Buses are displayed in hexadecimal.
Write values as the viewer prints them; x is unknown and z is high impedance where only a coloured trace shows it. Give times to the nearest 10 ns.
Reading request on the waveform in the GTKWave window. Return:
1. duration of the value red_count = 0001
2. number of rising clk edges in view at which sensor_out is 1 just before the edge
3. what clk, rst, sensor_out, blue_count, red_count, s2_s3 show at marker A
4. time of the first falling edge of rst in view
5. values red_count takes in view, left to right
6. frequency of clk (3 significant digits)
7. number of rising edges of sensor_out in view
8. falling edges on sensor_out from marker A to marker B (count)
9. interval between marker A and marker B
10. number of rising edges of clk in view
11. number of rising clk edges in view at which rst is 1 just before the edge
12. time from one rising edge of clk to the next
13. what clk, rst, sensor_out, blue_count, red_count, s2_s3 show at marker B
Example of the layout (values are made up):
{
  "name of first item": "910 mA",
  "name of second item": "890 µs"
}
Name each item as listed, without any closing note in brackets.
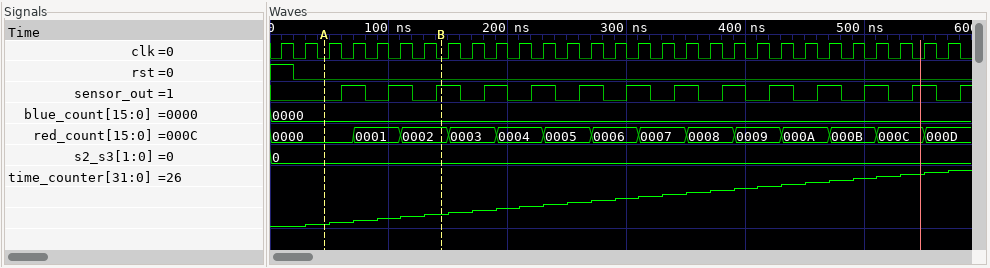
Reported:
{
  "duration of the value red_count = 0001": "40 ns",
  "number of rising clk edges in view at which sensor_out is 1 just before the edge": "13",
  "what clk, rst, sensor_out, blue_count, red_count, s2_s3 show at marker A": "clk=0, rst=0, sensor_out=0, blue_count=0000, red_count=0000, s2_s3=0",
  "time of the first falling edge of rst in view": "20 ns",
  "values red_count takes in view, left to right": "0000, 0001, 0002, 0003, 0004, 0005, 0006, 0007, 0008, 0009, 000A, 000B, 000C, 000D",
  "frequency of clk": "50.0 MHz",
  "number of rising edges of sensor_out in view": "14",
  "falling edges on sensor_out from marker A to marker B": "2",
  "interval between marker A and marker B": "100 ns",
  "number of rising edges of clk in view": "29",
  "number of rising clk edges in view at which rst is 1 just before the edge": "1",
  "time from one rising edge of clk to the next": "20 ns",
  "what clk, rst, sensor_out, blue_count, red_count, s2_s3 show at marker B": "clk=0, rst=0, sensor_out=1, blue_count=0000, red_count=0002, s2_s3=0"
}
